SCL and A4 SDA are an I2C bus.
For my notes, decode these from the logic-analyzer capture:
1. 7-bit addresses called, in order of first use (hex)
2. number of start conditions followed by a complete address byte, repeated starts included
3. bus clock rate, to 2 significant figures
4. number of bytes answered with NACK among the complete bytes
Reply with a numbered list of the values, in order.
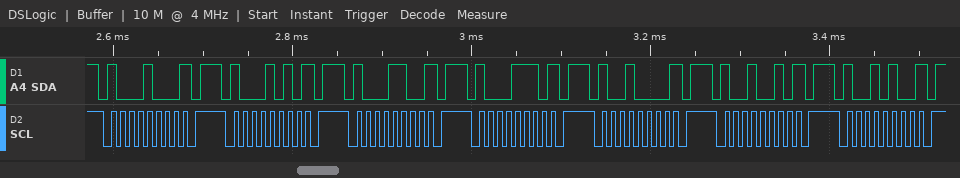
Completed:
1. 0x44 0x45 0x46 0x47 0x48 0x49 0x4A
2. 7
3. 100 kHz
4. 7
